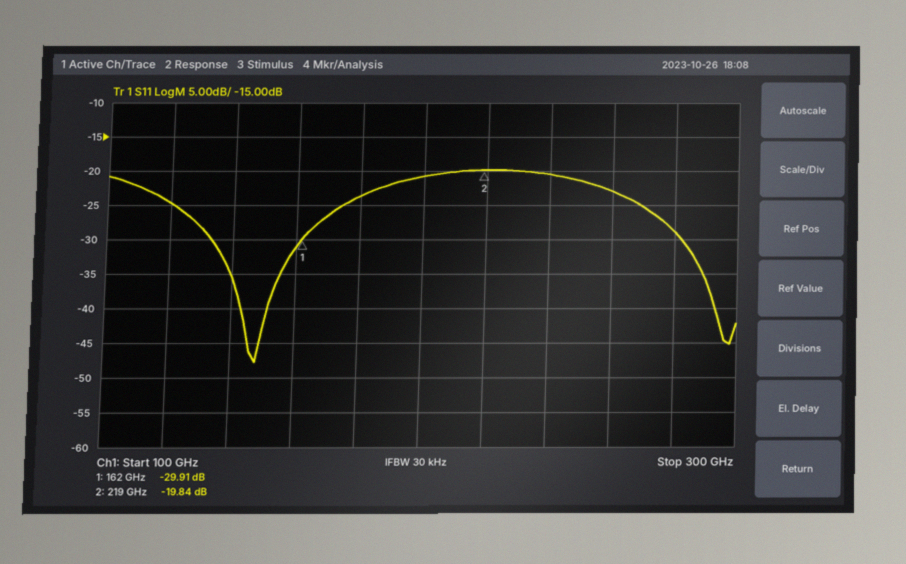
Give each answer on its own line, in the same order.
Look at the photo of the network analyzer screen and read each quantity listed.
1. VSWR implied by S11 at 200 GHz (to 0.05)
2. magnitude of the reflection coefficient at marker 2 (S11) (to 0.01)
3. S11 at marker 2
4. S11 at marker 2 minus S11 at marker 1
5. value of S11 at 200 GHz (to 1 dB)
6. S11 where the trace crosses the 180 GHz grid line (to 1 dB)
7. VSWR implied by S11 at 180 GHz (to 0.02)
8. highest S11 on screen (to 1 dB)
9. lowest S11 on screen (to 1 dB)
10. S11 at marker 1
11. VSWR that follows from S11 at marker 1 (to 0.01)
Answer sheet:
1.20
0.10
-19.84 dB
10.07 dB
-21 dB
-24 dB
1.14
-20 dB
-48 dB
-29.91 dB
1.07
